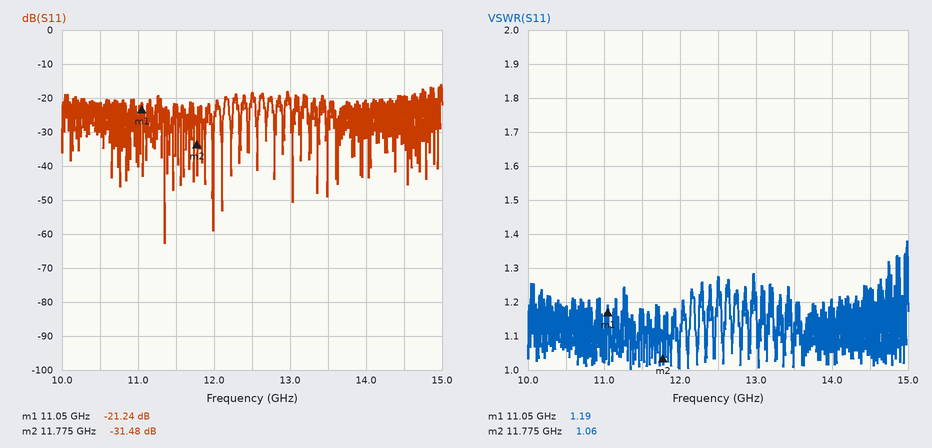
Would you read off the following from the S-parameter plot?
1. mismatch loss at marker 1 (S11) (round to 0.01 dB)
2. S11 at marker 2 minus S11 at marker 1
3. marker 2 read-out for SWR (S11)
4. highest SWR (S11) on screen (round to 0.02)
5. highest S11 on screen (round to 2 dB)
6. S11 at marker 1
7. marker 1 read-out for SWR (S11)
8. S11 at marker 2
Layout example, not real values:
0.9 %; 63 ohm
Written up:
0.03 dB; -10.24 dB; 1.06; 1.38; -16 dB; -21.24 dB; 1.19; -31.48 dB
